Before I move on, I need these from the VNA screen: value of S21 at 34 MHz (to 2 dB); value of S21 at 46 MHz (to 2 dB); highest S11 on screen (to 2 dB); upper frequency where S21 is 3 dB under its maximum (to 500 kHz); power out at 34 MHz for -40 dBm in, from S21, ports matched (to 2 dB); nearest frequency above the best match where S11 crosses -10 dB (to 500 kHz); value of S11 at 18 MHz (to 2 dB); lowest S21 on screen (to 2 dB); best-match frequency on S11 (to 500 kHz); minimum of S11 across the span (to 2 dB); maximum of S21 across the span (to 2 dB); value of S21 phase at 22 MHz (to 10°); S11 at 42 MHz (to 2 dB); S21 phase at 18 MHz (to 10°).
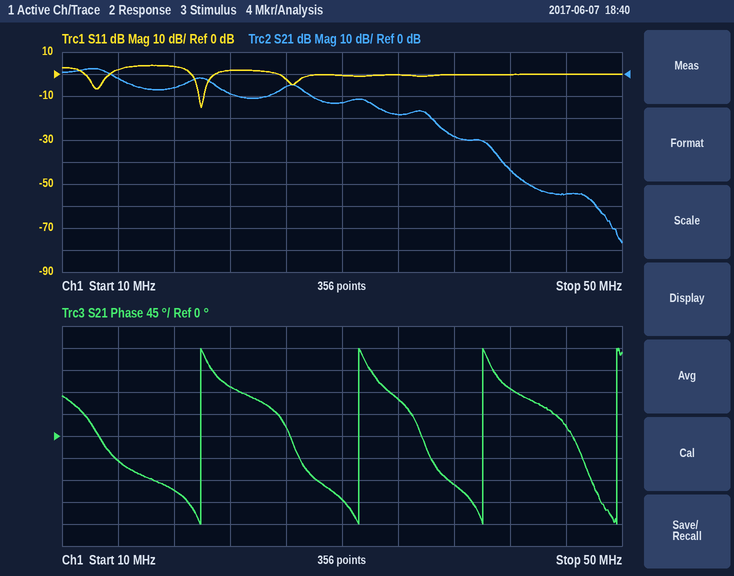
-18 dB
-54 dB
4 dB
13.5 MHz
-58 dBm
20.0 MHz
4 dB
-76 dB
20.0 MHz
-16 dB
2 dB
100°
0 dB
-110°
